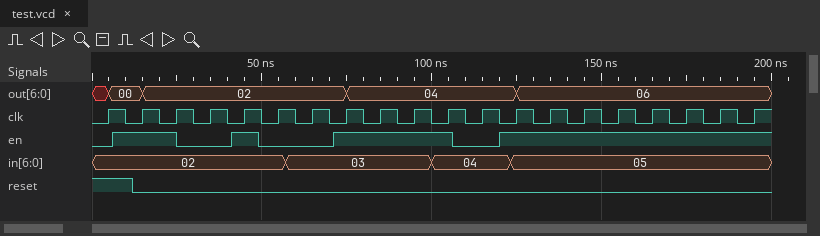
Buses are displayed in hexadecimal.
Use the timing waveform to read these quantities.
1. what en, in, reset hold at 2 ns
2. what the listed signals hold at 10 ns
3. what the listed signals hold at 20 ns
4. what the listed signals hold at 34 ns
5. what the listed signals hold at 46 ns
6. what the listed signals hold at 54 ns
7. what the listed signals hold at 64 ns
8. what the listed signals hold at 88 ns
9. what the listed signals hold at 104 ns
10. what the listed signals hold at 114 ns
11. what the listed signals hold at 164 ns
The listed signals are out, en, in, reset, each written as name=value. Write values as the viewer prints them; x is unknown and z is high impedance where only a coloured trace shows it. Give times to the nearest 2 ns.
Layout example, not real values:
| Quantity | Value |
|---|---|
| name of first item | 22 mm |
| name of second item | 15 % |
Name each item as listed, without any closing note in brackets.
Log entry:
| Quantity | Value |
|---|---|
| what en, in, reset hold at 2 ns | en=0, in=02, reset=1 |
| what the listed signals hold at 10 ns | out=00, en=1, in=02, reset=1 |
| what the listed signals hold at 20 ns | out=02, en=1, in=02, reset=0 |
| what the listed signals hold at 34 ns | out=02, en=0, in=02, reset=0 |
| what the listed signals hold at 46 ns | out=02, en=1, in=02, reset=0 |
| what the listed signals hold at 54 ns | out=02, en=0, in=02, reset=0 |
| what the listed signals hold at 64 ns | out=02, en=0, in=03, reset=0 |
| what the listed signals hold at 88 ns | out=04, en=1, in=03, reset=0 |
| what the listed signals hold at 104 ns | out=04, en=1, in=04, reset=0 |
| what the listed signals hold at 114 ns | out=04, en=0, in=04, reset=0 |
| what the listed signals hold at 164 ns | out=06, en=1, in=05, reset=0 |
